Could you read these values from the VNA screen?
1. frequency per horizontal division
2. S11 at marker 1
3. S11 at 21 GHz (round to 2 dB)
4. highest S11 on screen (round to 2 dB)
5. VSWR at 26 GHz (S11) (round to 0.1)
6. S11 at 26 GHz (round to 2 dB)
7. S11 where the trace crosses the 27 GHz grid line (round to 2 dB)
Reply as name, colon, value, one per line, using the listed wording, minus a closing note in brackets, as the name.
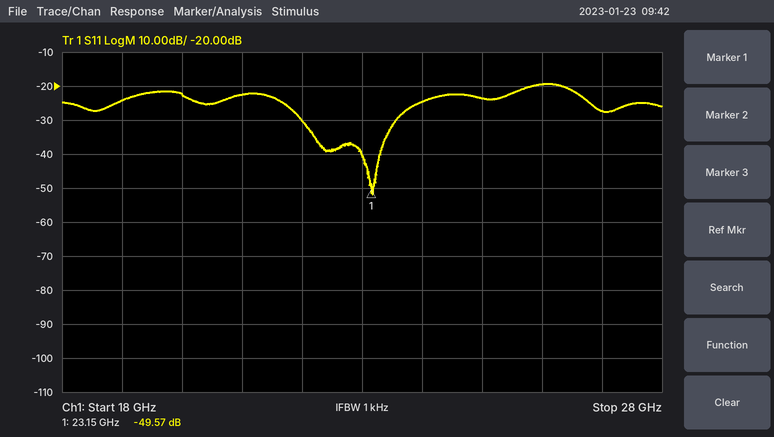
frequency per horizontal division: 1 GHz
S11 at marker 1: -49.57 dB
S11 at 21 GHz: -22 dB
highest S11 on screen: -20 dB
VSWR at 26 GHz (S11): 1.2
S11 at 26 GHz: -20 dB
S11 where the trace crosses the 27 GHz grid line: -28 dB
